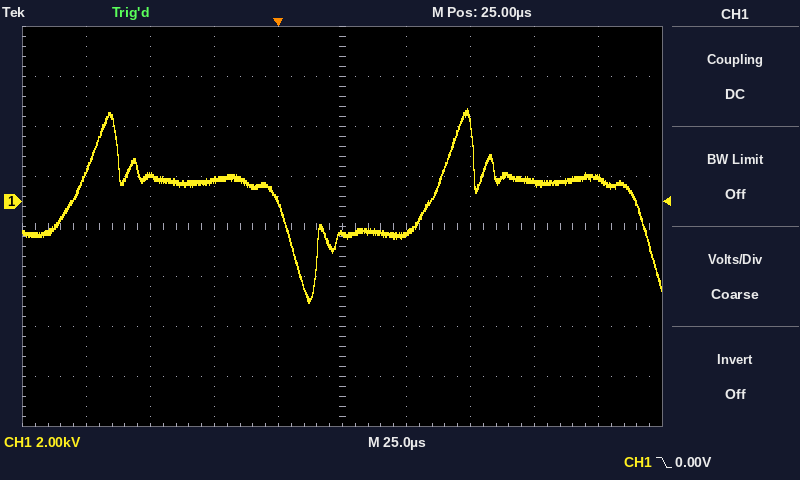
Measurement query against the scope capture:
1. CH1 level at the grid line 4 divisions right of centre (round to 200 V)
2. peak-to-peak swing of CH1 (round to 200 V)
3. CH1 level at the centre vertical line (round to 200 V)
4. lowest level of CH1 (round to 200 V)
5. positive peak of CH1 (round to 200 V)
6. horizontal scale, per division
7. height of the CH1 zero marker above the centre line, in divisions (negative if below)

1.0 kV
7.8 kV
-1.2 kV
-4.0 kV
3.8 kV
25 µs
+0.5 div
